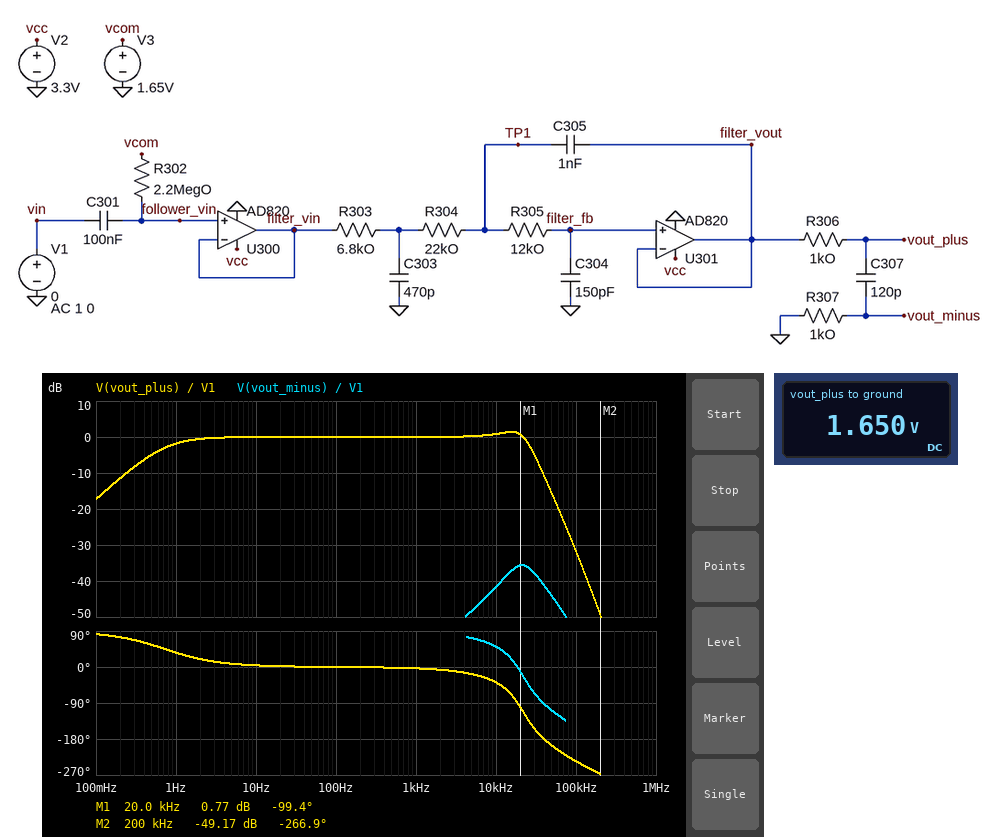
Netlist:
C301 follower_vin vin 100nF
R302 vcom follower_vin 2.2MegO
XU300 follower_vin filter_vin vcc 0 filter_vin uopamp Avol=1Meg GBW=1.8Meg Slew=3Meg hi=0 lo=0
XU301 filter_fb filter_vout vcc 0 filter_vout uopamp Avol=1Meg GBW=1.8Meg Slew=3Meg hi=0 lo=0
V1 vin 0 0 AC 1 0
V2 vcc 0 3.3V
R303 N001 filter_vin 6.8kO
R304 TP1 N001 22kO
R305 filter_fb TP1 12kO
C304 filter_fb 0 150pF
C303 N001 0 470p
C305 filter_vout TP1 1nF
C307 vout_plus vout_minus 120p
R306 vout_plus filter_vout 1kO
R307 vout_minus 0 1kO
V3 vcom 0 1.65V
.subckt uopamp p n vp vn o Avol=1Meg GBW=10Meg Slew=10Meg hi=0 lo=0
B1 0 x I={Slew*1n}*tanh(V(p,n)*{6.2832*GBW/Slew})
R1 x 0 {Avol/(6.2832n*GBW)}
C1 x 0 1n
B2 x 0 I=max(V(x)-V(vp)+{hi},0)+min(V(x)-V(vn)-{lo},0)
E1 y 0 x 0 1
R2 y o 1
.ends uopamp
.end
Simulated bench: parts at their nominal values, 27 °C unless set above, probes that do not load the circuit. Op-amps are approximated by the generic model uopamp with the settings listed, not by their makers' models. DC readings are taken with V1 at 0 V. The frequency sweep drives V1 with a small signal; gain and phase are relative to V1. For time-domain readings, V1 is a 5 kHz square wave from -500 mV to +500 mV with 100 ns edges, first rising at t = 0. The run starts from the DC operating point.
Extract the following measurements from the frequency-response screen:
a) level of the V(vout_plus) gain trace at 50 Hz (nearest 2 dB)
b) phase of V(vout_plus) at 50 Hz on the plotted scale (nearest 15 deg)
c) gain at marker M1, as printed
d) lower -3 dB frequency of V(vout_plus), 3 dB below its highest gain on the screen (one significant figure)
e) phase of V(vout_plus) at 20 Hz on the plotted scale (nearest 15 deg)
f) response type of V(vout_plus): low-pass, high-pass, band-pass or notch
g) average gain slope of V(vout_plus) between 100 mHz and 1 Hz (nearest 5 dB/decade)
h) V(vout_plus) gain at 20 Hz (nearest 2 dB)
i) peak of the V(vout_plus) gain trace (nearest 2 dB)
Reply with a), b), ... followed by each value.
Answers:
a) 0 dB
b) 0 deg
c) 0.77 dB
d) 1 Hz
e) 0 deg
f) band-pass
g) 15 dB/decade
h) 0 dB
i) 2 dB
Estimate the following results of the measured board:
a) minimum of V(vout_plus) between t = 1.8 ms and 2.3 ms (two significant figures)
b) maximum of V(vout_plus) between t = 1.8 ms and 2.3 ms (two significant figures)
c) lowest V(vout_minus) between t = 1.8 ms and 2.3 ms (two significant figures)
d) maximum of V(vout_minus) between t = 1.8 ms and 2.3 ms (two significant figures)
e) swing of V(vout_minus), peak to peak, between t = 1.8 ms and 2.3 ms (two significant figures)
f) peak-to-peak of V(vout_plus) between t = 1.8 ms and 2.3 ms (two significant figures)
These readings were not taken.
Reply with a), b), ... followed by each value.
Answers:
a) 1.5 V
b) 2.8 V
c) -8.7 mV
d) 8.7 mV
e) 17 mV
f) 1.4 V
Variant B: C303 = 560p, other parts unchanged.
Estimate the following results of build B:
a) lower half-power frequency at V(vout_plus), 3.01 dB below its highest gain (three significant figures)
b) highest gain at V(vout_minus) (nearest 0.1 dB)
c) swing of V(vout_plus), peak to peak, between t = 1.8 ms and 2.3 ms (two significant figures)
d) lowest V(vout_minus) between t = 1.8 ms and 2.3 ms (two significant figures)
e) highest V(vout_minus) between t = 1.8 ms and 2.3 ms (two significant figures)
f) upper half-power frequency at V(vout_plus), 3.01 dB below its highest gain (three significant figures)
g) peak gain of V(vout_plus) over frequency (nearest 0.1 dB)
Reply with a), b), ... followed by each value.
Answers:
a) 995 mHz
b) -35.9 dB
c) 1.3 V
d) -8.4 mV
e) 8.4 mV
f) 24.8 kHz
g) 1.2 dB
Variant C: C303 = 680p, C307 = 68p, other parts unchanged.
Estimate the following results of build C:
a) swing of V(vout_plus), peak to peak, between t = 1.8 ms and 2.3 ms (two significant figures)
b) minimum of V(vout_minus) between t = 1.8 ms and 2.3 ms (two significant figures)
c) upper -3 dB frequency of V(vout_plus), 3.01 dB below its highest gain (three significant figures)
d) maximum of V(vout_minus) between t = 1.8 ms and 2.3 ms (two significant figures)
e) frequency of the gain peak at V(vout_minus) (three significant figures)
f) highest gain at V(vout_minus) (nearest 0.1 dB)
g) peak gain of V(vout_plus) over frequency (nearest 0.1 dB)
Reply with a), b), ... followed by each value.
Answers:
a) 1.3 V
b) -4.6 mV
c) 24.5 kHz
d) 4.6 mV
e) 21.1 kHz
f) -41.3 dB
g) 0.9 dB
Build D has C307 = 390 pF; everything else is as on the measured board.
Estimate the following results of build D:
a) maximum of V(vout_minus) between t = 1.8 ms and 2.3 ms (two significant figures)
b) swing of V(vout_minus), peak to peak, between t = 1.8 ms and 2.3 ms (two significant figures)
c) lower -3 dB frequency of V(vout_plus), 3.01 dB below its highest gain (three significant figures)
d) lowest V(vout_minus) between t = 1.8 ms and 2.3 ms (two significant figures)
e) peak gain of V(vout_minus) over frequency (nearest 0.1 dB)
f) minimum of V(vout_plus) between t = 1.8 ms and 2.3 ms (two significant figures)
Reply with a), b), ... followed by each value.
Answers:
a) 28 mV
b) 56 mV
c) 1.07 Hz
d) -28 mV
e) -25.4 dB
f) 1.5 V
